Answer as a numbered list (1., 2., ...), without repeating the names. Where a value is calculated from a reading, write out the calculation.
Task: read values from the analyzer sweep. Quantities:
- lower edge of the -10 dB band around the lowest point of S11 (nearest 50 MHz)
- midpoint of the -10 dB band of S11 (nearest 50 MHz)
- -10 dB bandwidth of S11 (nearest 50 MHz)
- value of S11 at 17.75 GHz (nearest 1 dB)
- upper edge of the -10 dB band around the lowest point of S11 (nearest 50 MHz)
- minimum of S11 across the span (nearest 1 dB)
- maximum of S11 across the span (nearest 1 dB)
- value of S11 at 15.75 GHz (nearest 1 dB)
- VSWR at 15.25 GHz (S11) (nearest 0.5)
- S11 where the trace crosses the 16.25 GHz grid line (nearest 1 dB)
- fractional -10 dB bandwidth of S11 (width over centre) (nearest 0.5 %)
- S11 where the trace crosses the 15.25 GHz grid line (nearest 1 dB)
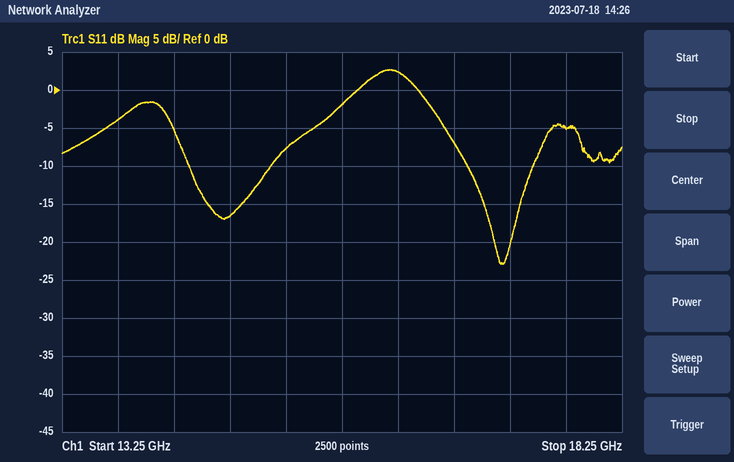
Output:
1. 16.85 GHz
2. 17.15 GHz
3. 17.45 GHz − 16.85 GHz = 600 MHz
4. -5 dB
5. 17.45 GHz
6. -23 dB
7. 3 dB
8. -2 dB
9. |Γ| = 10^(-8/20) = 0.3981; VSWR = (1 + 0.3981)/(1 − 0.3981) ≈ 2.32, so 2.5 to the nearest 0.5
10. 2 dB
11. 600 MHz / 17.15 GHz ≈ 3.5 %
12. -8 dB
